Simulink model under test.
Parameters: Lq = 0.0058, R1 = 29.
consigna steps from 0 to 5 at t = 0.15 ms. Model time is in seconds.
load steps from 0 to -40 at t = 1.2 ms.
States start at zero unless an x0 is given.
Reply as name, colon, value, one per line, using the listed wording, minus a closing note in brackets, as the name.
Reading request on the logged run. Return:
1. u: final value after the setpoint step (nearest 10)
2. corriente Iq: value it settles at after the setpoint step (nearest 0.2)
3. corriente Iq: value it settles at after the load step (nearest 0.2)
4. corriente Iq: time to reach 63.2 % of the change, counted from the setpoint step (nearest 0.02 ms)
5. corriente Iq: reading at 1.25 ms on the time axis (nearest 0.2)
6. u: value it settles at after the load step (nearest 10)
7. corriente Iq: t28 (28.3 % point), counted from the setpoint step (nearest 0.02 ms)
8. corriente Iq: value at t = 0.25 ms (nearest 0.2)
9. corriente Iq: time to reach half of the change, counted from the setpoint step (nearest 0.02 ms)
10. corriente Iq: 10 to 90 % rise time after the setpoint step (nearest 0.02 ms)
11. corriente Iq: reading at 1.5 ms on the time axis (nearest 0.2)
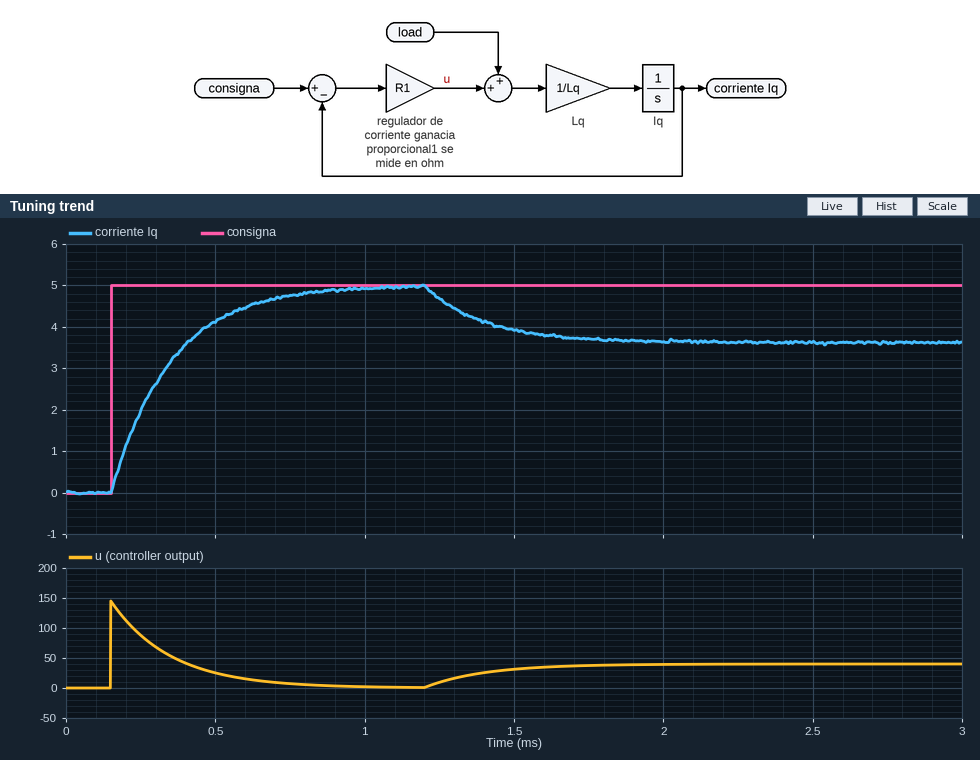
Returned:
u: final value after the setpoint step: 0
corriente Iq: value it settles at after the setpoint step: 5.0
corriente Iq: value it settles at after the load step: 3.6
corriente Iq: time to reach 63.2 % of the change, counted from the setpoint step: 0.20 ms
corriente Iq: reading at 1.25 ms on the time axis: 4.6
u: value it settles at after the load step: 40
corriente Iq: t28 (28.3 % point), counted from the setpoint step: 0.06 ms
corriente Iq: value at t = 0.25 ms: 2.0
corriente Iq: time to reach half of the change, counted from the setpoint step: 0.14 ms
corriente Iq: 10 to 90 % rise time after the setpoint step: 0.44 ms
corriente Iq: reading at 1.5 ms on the time axis: 4.0
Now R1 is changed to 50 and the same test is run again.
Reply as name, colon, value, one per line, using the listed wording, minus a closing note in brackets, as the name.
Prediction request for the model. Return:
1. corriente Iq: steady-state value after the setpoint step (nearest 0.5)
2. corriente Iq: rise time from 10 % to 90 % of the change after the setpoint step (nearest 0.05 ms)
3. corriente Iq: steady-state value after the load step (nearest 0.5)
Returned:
corriente Iq: steady-state value after the setpoint step: 5.0
corriente Iq: rise time from 10 % to 90 % of the change after the setpoint step: 0.25 ms
corriente Iq: steady-state value after the load step: 4.0
